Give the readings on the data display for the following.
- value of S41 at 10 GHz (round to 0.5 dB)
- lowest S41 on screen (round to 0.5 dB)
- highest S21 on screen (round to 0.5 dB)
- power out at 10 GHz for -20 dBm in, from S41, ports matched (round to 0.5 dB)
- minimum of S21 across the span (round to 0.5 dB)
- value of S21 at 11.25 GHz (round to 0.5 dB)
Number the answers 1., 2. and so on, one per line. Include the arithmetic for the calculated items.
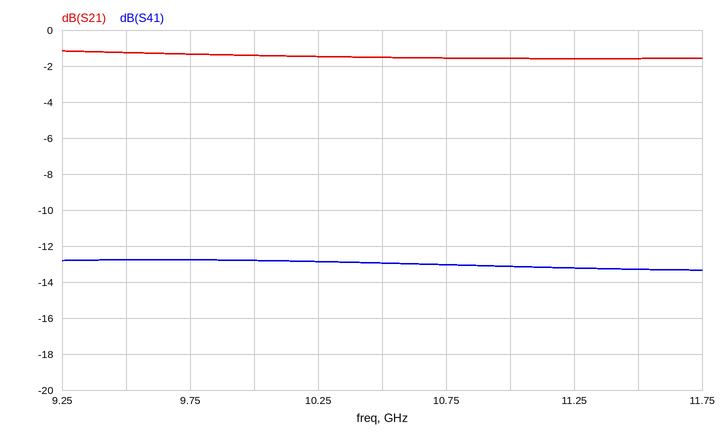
1. -13.0 dB
2. -13.5 dB
3. -1.0 dB
4. -20 dBm + (-13.0 dB) = -33.0 dBm
5. -1.5 dB
6. -1.5 dB
